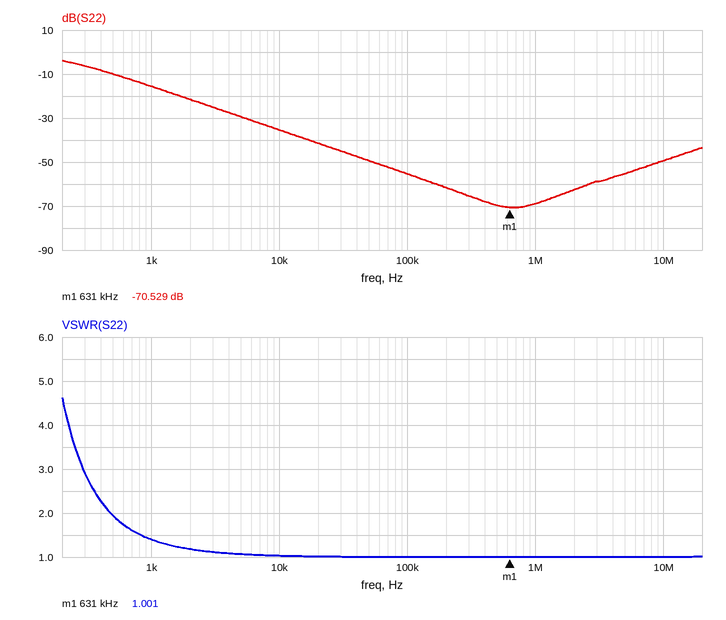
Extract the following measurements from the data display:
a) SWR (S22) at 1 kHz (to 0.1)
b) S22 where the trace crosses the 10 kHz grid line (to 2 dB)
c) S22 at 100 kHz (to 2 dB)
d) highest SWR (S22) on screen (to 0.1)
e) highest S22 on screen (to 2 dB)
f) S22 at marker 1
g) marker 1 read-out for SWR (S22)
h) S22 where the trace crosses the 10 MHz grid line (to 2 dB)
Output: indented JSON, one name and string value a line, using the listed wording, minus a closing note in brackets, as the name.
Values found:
{
  "SWR (S22) at 1 kHz": "1.4",
  "S22 where the trace crosses the 10 kHz grid line": "-36 dB",
  "S22 at 100 kHz": "-56 dB",
  "highest SWR (S22) on screen": "4.6",
  "highest S22 on screen": "-4 dB",
  "S22 at marker 1": "-70.529 dB",
  "marker 1 read-out for SWR": "1.001",
  "S22 where the trace crosses the 10 MHz grid line": "-50 dB"
}
